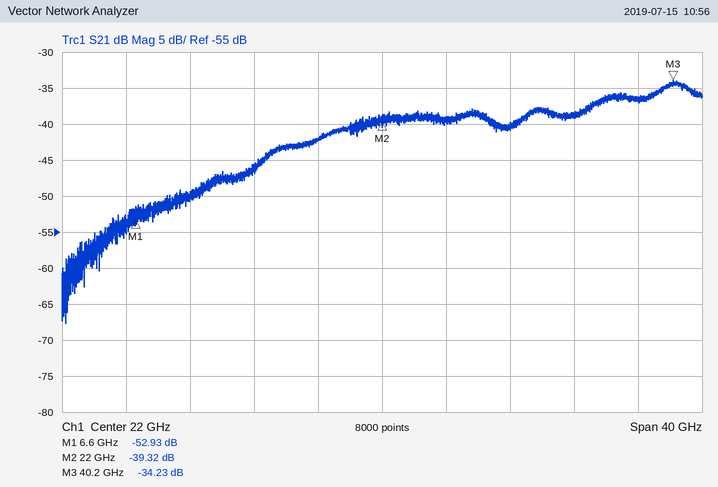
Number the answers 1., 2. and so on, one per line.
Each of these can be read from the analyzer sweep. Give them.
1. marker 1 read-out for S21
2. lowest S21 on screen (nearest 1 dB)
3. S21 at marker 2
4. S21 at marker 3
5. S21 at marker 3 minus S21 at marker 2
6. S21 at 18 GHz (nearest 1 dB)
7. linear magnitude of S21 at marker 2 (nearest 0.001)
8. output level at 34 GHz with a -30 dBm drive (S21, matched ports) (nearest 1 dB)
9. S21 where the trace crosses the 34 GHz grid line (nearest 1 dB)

1. -52.93 dB
2. -68 dB
3. -39.32 dB
4. -34.23 dB
5. 5.09 dB
6. -42 dB
7. 0.011
8. -69 dBm
9. -39 dB
